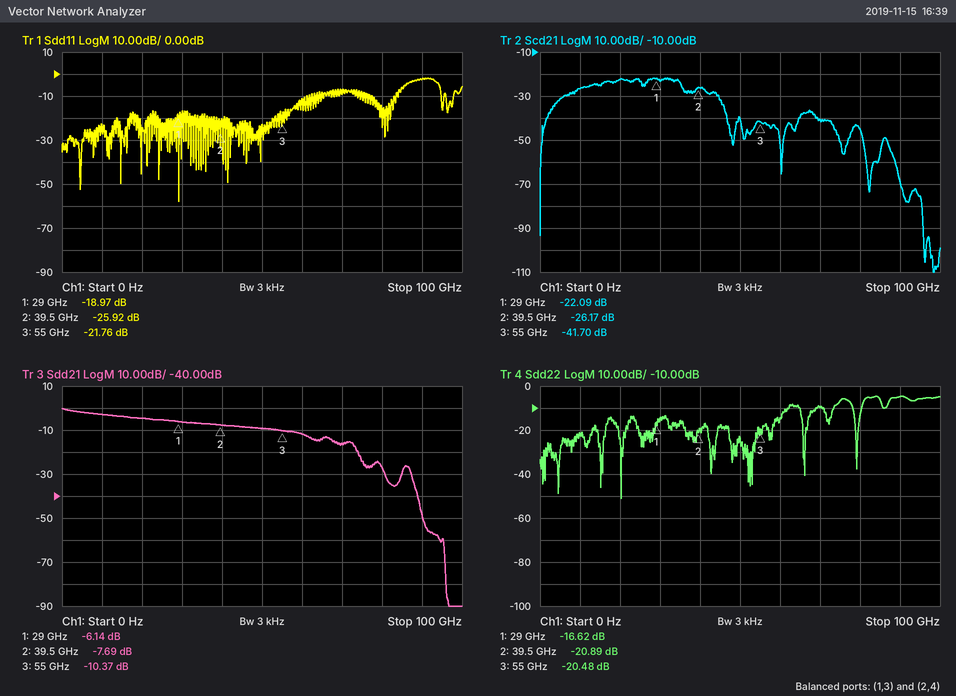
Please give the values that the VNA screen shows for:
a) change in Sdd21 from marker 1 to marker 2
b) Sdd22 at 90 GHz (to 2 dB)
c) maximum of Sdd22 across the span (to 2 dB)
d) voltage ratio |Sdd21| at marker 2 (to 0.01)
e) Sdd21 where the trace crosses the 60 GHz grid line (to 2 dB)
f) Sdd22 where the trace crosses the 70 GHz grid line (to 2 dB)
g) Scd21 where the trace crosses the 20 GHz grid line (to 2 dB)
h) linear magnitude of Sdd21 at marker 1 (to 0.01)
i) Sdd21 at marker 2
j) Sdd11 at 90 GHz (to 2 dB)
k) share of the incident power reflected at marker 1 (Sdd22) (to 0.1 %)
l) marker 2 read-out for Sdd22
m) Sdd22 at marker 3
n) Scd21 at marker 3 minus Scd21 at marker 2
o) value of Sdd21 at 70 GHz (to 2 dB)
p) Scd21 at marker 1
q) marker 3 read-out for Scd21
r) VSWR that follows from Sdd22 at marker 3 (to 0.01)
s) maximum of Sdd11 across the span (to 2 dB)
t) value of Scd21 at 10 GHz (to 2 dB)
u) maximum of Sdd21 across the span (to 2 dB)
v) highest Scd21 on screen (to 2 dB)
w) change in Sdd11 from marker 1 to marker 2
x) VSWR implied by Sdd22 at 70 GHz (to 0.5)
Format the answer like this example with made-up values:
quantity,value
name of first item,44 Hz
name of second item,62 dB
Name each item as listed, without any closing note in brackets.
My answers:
quantity,value
change in Sdd21 from marker 1 to marker 2,-1.55 dB
Sdd22 at 90 GHz,-4 dB
maximum of Sdd22 across the span,-4 dB
voltage ratio |Sdd21| at marker 2,0.41
Sdd21 where the trace crosses the 60 GHz grid line,-12 dB
Sdd22 where the trace crosses the 70 GHz grid line,-10 dB
Scd21 where the trace crosses the 20 GHz grid line,-22 dB
linear magnitude of Sdd21 at marker 1,0.49
Sdd21 at marker 2,-7.69 dB
Sdd11 at 90 GHz,-2 dB
share of the incident power reflected at marker 1 (Sdd22),2.2 %
marker 2 read-out for Sdd22,-20.89 dB
Sdd22 at marker 3,-20.48 dB
Scd21 at marker 3 minus Scd21 at marker 2,-15.53 dB
value of Sdd21 at 70 GHz,-16 dB
Scd21 at marker 1,-22.09 dB
marker 3 read-out for Scd21,-41.70 dB
VSWR that follows from Sdd22 at marker 3,1.21
maximum of Sdd11 across the span,-2 dB
value of Scd21 at 10 GHz,-26 dB
maximum of Sdd21 across the span,0 dB
highest Scd21 on screen,-22 dB
change in Sdd11 from marker 1 to marker 2,-6.95 dB
VSWR implied by Sdd22 at 70 GHz,2.0
